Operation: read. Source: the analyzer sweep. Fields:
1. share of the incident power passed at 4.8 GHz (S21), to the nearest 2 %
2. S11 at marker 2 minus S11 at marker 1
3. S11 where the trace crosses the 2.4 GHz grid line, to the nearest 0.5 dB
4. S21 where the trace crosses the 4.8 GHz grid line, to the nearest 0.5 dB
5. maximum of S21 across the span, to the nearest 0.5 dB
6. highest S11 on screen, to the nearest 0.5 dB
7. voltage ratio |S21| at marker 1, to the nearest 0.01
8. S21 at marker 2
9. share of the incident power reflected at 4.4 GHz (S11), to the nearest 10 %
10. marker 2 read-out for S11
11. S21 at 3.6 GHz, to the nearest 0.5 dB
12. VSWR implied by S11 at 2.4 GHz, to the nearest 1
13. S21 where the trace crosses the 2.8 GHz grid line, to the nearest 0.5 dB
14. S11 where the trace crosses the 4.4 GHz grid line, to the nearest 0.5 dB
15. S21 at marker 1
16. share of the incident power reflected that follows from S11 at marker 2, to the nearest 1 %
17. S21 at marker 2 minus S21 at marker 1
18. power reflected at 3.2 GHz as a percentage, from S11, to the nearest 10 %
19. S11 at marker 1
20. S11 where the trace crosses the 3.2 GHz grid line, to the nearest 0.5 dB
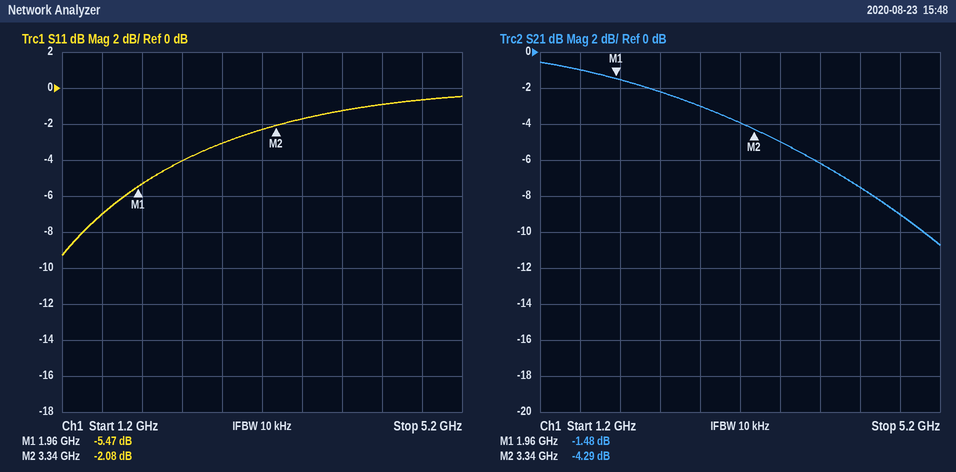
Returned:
12 %
3.39 dB
-4.0 dB
-9.0 dB
-0.5 dB
-0.5 dB
0.84
-4.29 dB
80 %
-2.08 dB
-5.0 dB
4
-3.0 dB
-1.0 dB
-1.48 dB
62 %
-2.81 dB
60 %
-5.47 dB
-2.5 dB
